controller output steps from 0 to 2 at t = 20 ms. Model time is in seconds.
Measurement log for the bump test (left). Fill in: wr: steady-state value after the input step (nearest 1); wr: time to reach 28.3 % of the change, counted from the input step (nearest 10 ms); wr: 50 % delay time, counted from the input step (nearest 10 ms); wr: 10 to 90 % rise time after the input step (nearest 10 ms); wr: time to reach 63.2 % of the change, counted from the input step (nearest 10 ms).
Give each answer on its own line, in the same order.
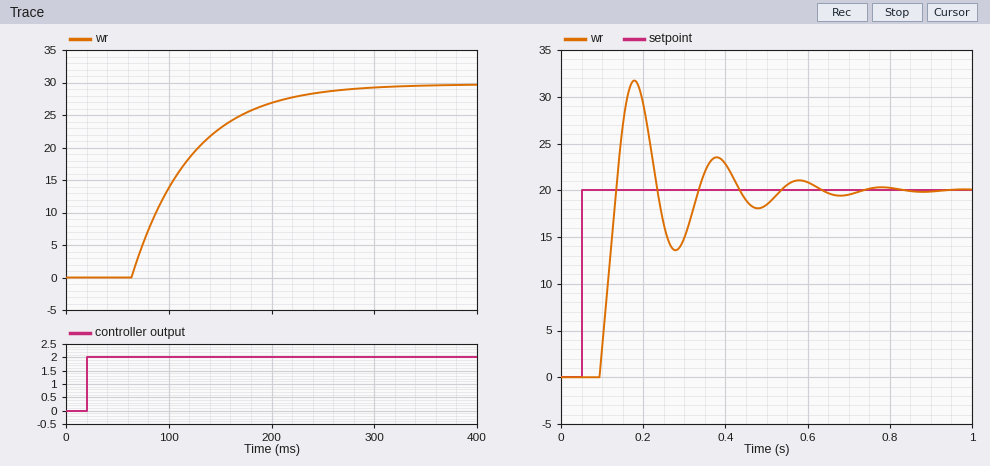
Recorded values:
30
60 ms
80 ms
130 ms
100 ms
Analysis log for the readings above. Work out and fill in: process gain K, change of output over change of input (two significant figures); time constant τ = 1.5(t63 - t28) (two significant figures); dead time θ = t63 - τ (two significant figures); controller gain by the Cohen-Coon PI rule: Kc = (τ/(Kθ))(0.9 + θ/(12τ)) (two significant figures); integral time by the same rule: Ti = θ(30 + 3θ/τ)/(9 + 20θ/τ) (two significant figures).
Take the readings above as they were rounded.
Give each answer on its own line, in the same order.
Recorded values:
15
60 ms
40 ms
0.096
57 ms
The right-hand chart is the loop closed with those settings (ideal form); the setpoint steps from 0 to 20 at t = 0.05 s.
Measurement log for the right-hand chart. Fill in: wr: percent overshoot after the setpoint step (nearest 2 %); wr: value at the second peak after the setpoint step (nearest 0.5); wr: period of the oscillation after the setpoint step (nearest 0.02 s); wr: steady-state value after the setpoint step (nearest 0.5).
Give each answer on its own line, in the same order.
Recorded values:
58 %
23.5
0.20 s
20.0
